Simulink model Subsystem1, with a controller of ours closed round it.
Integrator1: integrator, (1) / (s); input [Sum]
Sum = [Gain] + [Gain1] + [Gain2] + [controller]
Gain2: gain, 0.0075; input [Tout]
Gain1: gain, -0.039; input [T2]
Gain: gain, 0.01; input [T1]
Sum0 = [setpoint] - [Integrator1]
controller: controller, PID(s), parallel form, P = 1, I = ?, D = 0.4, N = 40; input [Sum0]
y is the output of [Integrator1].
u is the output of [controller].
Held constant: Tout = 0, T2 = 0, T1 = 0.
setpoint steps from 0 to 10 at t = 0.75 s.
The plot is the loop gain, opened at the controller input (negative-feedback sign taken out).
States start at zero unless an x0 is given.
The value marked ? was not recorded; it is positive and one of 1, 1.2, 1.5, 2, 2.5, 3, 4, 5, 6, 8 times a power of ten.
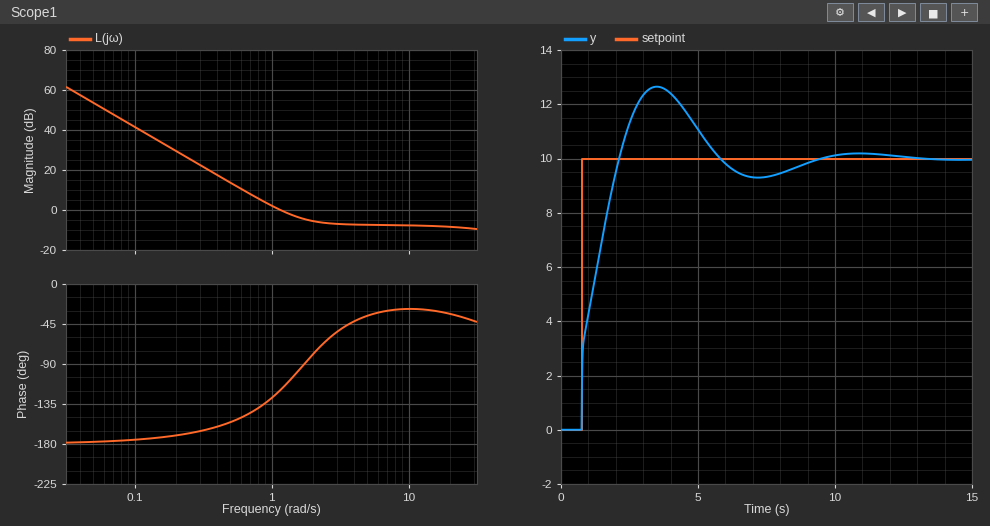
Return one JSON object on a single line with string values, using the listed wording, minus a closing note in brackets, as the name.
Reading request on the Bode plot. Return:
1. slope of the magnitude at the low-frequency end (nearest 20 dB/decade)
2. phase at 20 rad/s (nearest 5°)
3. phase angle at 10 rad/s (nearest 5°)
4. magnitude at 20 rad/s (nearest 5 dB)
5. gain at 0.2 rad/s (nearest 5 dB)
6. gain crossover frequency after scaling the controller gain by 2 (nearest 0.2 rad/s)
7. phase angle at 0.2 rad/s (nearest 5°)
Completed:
{"slope of the magnitude at the low-frequency end": "-40 dB/decade", "phase at 20 rad/s": "-35°", "phase angle at 10 rad/s": "-30°", "magnitude at 20 rad/s": "-10 dB", "gain at 0.2 rad/s": "30 dB", "gain crossover frequency after scaling the controller gain by 2": "2.2 rad/s", "phase angle at 0.2 rad/s": "-170°"}
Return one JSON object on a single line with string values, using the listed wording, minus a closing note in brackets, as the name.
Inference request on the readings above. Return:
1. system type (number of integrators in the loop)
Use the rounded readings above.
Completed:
{"system type": "2"}
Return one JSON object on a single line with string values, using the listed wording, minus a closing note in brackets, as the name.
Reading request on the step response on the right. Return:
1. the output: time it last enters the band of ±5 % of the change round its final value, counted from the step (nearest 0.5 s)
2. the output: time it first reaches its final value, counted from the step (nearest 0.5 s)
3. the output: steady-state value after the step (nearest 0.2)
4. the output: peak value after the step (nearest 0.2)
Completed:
{"the output: time it last enters the band of ±5 % of the change round its final value, counted from the step": "7.5 s", "the output: time it first reaches its final value, counted from the step": "1.5 s", "the output: steady-state value after the step": "10.0", "the output: peak value after the step": "12.6"}
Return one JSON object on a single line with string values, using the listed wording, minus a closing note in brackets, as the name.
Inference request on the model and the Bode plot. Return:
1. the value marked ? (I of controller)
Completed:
{"the value marked ?": "1.2"}
